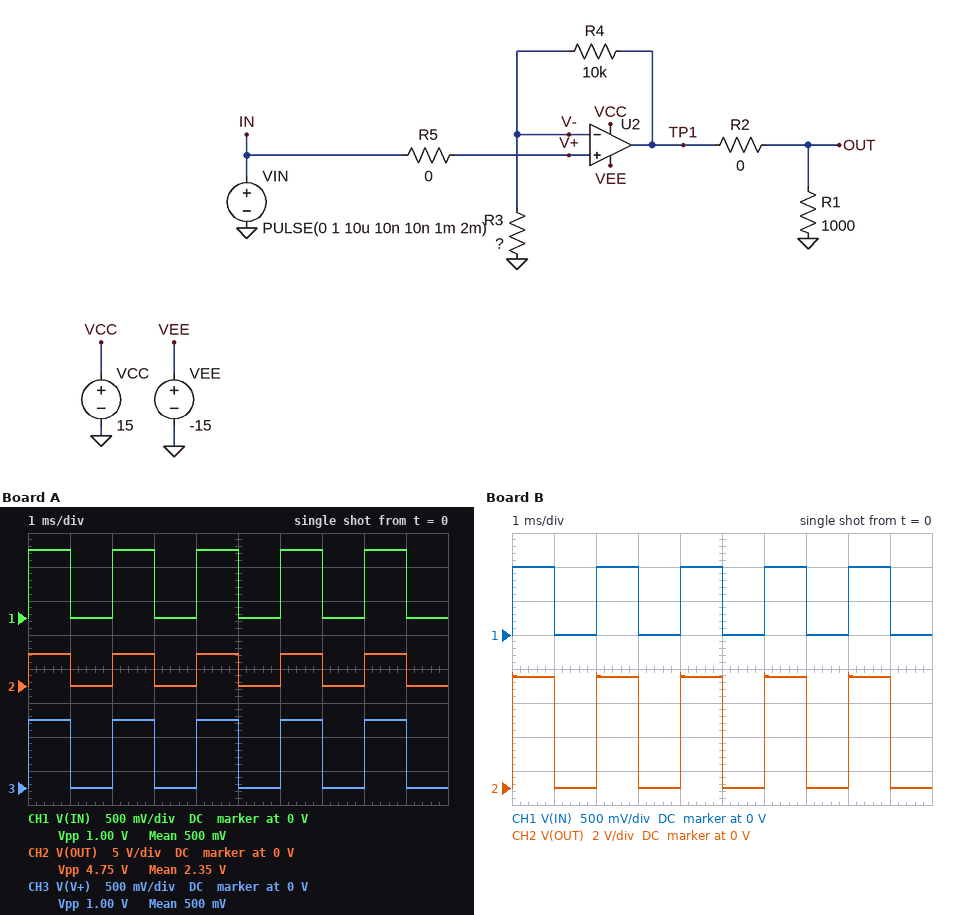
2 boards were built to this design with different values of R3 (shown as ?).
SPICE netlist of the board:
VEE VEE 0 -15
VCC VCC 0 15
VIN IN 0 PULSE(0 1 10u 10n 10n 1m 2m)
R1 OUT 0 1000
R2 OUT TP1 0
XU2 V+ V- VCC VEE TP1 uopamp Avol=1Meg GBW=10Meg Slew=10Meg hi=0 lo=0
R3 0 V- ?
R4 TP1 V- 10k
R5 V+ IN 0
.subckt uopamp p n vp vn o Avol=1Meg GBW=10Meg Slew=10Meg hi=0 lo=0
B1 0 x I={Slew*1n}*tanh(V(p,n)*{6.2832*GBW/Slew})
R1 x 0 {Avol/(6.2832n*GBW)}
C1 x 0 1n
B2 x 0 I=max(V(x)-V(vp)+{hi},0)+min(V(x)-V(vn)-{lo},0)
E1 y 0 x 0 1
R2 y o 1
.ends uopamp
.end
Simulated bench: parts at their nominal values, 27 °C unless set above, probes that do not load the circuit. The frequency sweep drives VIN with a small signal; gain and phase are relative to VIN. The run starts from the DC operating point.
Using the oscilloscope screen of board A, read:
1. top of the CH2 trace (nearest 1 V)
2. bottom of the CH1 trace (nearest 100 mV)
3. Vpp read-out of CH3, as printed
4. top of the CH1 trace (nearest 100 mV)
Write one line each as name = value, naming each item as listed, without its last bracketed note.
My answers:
top of the CH2 trace = 5 V
bottom of the CH1 trace = 0 V
Vpp read-out of CH3, as printed = 1.00 V
top of the CH1 trace = 1.0 V
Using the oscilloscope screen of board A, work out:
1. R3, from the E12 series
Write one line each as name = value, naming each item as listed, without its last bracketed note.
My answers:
R3, from the E12 series = 2.7 kΩ
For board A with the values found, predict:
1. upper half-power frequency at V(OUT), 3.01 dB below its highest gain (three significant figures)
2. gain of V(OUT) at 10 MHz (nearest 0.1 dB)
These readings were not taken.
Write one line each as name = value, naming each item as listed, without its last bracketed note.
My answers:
upper half-power frequency at V(OUT), 3.01 dB below its highest gain = 2.12 MHz
gain of V(OUT) at 10 MHz = -0.2 dB
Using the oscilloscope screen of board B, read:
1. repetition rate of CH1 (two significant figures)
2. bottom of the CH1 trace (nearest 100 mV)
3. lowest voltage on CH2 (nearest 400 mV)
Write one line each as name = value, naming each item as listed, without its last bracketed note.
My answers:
repetition rate of CH1 = 500 Hz
bottom of the CH1 trace = 0 V
lowest voltage on CH2 = 0 V
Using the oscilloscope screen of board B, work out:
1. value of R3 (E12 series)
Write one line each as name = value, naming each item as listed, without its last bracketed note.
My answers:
value of R3 = 1.8 kΩ
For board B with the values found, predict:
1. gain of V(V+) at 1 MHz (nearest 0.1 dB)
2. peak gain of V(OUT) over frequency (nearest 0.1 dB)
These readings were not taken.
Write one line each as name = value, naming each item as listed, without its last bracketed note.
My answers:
gain of V(V+) at 1 MHz = 0 dB
peak gain of V(OUT) over frequency = 16.3 dB
